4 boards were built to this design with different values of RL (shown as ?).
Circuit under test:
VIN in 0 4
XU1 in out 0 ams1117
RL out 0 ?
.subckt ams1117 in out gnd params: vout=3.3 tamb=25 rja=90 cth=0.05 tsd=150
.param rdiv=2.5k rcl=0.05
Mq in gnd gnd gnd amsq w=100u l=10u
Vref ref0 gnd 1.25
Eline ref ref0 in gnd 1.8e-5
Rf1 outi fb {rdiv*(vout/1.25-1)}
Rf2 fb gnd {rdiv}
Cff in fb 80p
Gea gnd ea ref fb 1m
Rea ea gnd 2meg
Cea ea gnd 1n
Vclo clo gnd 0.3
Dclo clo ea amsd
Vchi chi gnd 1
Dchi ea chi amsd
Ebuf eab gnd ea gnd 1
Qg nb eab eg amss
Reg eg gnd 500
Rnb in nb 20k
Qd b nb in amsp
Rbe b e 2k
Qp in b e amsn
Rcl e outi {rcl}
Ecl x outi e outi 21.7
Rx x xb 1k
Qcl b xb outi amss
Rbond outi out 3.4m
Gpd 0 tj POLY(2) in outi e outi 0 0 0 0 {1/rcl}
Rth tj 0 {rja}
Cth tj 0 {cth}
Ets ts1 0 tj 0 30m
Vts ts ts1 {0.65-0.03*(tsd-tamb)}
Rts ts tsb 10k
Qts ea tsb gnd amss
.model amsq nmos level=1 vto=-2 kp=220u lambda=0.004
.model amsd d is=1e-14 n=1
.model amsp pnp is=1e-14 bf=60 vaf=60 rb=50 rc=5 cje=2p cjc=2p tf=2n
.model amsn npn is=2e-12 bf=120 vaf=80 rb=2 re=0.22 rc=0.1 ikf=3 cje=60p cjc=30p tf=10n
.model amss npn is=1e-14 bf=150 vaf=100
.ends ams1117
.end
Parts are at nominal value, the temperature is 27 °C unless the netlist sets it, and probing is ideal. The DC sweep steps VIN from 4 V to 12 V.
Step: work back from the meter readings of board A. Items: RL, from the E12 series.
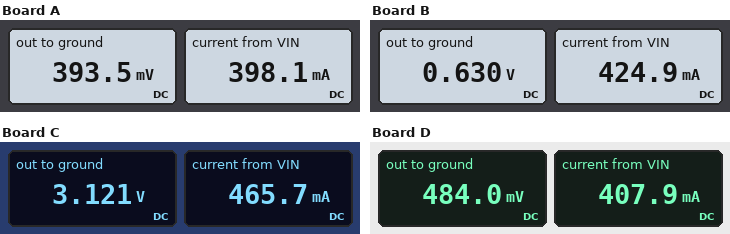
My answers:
1 Ω
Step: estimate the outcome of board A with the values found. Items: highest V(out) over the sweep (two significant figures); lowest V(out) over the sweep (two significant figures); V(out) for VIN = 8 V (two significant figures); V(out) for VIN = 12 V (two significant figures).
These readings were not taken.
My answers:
390 mV
120 mV
180 mV
120 mV
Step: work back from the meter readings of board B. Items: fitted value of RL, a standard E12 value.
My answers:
1.5 Ω
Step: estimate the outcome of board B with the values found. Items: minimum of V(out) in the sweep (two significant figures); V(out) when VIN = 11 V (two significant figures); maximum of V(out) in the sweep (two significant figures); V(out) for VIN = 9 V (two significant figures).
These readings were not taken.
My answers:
180 mV
200 mV
630 mV
240 mV
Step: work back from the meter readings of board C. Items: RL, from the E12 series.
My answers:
6.8 Ω
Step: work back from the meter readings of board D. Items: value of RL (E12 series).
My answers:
1.2 Ω
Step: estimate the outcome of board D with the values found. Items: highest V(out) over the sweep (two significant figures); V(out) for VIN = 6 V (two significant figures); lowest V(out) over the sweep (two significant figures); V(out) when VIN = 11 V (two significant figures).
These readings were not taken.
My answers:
480 mV
300 mV
140 mV
160 mV
